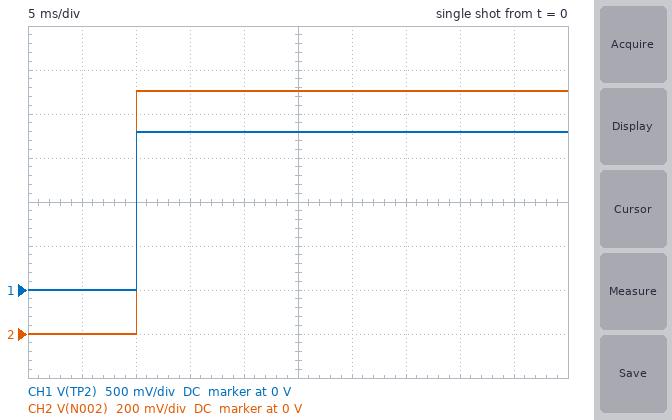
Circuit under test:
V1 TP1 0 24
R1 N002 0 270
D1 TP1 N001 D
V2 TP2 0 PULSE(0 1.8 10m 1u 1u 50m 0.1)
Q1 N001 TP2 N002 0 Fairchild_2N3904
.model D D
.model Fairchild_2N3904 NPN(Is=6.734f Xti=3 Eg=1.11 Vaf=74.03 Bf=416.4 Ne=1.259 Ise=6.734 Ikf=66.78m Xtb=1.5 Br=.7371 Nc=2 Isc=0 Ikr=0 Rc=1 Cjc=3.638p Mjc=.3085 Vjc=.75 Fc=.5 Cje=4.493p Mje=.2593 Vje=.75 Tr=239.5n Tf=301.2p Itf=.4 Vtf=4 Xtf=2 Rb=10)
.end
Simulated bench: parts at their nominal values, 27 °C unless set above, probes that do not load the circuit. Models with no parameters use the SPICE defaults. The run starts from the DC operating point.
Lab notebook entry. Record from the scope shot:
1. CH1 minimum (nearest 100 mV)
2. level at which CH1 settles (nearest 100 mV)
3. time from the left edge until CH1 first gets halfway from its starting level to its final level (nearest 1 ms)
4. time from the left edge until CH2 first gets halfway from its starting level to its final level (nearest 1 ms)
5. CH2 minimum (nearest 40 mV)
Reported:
0 V
1.8 V
10 ms
10 ms
0 V
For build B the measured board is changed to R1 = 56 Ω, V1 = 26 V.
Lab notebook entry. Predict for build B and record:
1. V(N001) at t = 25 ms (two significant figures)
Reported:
25 V
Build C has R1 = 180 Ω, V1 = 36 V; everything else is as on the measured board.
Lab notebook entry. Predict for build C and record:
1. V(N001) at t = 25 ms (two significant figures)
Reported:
35 V
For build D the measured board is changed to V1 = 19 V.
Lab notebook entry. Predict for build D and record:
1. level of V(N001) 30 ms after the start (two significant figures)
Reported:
18 V
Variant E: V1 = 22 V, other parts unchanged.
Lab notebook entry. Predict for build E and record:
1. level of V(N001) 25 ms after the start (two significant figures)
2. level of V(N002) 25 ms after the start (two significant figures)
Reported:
21 V
1.1 V
